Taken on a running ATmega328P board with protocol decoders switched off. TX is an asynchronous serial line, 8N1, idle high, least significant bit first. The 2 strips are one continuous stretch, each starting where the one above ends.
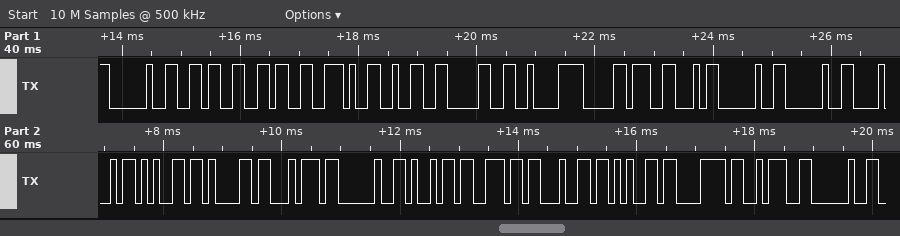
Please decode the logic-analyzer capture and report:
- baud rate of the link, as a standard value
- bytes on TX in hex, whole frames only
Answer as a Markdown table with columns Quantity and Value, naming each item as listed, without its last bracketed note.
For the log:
| Quantity | Value |
|---|---|
| baud rate of the link, as a standard value | 9600 baud |
| bytes on TX in hex, whole frames only | 20 36 36 2E 32 30 C2 B0 46 20 20 48 65 61 74 20 69 6E 64 65 78 3A 20 |
